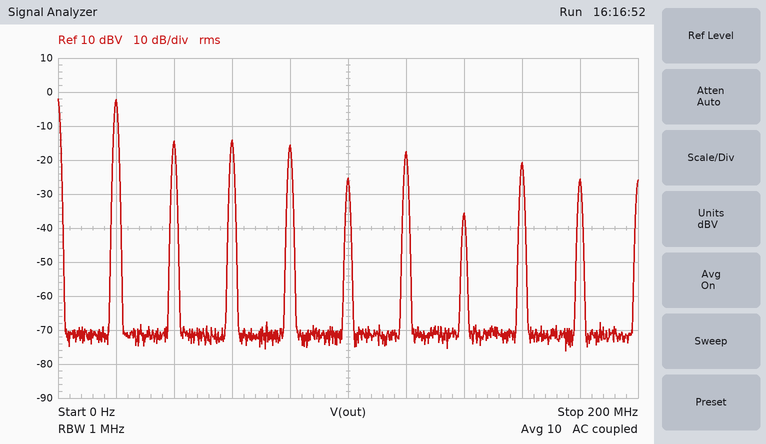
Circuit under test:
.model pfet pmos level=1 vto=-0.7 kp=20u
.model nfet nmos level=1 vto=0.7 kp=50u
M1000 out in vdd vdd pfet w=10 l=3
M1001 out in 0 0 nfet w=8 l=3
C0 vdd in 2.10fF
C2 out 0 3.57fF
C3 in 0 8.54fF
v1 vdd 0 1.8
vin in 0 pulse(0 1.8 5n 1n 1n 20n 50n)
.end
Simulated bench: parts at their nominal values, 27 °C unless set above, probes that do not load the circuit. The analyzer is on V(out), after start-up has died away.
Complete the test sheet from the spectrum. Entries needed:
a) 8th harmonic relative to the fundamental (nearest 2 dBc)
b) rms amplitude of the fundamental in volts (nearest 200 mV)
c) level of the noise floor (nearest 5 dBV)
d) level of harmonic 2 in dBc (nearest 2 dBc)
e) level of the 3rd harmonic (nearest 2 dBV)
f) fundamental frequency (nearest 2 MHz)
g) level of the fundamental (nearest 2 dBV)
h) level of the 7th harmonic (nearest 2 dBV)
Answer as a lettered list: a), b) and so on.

a) -18 dBc
b) 800 mV
c) -70 dBV
d) -12 dBc
e) -14 dBV
f) 20 MHz
g) -2 dBV
h) -36 dBV
